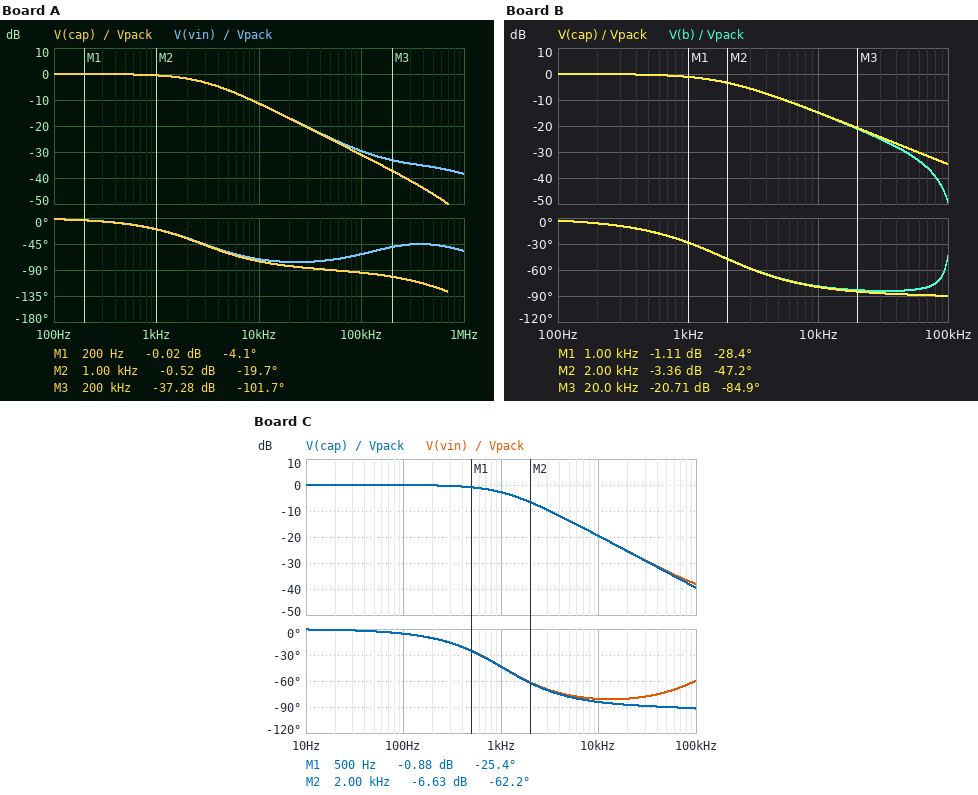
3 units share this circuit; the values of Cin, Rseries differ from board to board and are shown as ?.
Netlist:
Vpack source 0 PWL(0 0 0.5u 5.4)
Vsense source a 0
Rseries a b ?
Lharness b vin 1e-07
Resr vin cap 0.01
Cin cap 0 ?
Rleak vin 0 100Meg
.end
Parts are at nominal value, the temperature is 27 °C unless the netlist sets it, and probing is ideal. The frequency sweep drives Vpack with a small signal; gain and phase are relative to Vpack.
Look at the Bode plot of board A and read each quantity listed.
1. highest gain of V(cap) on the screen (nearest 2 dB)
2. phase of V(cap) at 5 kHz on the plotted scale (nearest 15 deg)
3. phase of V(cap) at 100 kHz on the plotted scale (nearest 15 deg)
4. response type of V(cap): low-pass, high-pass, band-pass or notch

0 dB
-60 deg
-90 deg
low-pass
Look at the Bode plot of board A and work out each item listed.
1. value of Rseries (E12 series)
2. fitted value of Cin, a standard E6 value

0.56 Ω
100 µF
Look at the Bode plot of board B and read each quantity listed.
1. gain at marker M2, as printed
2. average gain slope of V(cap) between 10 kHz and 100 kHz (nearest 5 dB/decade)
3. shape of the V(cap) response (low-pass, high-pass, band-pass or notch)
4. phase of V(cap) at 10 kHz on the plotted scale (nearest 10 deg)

-3.36 dB
-20 dB/decade
low-pass
-80 deg
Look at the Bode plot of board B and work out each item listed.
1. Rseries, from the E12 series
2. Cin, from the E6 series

3.9 Ω
22 µF
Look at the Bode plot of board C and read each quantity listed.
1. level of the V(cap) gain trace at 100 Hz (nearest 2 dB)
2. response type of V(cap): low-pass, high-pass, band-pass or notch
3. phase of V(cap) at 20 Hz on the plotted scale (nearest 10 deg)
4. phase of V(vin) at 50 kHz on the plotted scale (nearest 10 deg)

0 dB
low-pass
0 deg
-70 deg
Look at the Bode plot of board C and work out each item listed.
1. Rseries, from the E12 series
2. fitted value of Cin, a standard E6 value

1.5 Ω
100 µF
